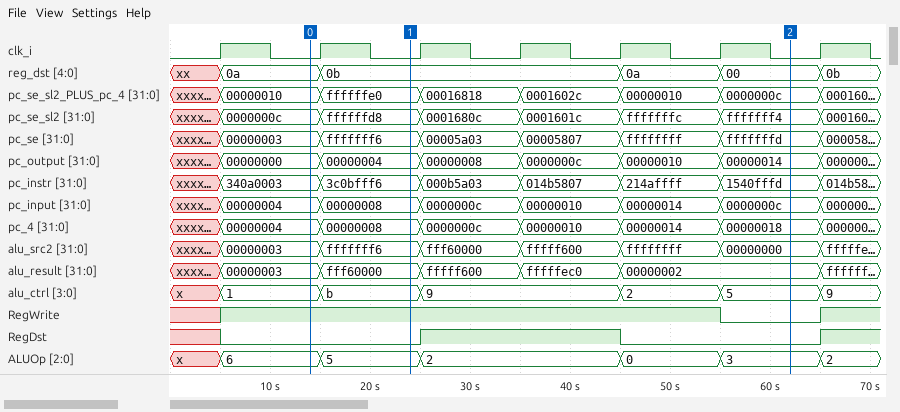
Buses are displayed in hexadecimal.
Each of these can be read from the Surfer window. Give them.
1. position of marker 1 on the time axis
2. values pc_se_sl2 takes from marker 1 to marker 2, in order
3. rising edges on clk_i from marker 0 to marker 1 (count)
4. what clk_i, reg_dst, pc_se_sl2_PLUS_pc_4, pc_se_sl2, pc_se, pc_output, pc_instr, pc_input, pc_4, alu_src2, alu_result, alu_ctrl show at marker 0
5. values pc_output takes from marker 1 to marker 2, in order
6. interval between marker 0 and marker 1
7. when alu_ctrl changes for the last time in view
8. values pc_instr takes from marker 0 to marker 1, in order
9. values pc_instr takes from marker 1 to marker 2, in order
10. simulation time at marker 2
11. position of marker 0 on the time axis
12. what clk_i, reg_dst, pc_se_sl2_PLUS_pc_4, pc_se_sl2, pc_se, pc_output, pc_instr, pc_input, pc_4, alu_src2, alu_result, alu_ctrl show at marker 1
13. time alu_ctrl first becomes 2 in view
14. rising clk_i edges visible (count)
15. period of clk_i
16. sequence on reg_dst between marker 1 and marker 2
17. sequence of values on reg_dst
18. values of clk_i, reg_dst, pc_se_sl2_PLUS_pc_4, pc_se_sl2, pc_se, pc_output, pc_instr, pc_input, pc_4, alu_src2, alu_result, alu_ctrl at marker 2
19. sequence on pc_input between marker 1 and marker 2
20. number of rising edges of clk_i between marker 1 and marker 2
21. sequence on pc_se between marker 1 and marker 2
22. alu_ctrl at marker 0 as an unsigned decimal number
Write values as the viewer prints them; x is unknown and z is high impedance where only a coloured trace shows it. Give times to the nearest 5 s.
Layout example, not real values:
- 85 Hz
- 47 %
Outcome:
- 25 s
- ffffffd8, 0001680c, 0001601c, fffffffc, fffffff4
- 1
- clk_i=0, reg_dst=0a, pc_se_sl2_PLUS_pc_4=00000010, pc_se_sl2=0000000c, pc_se=00000003, pc_output=00000000, pc_instr=340a0003, pc_input=00000004, pc_4=00000004, alu_src2=00000003, alu_result=00000003, alu_ctrl=1
- 00000004, 00000008, 0000000c, 00000010, 00000014
- 10 s
- 65 s
- 340a0003, 3c0bfff6
- 3c0bfff6, 000b5a03, 014b5807, 214affff, 1540fffd
- 60 s
- 15 s
- clk_i=0, reg_dst=0b, pc_se_sl2_PLUS_pc_4=ffffffe0, pc_se_sl2=ffffffd8, pc_se=fffffff6, pc_output=00000004, pc_instr=3c0bfff6, pc_input=00000008, pc_4=00000008, alu_src2=fffffff6, alu_result=fff60000, alu_ctrl=b
- 45 s
- 7
- 10 s
- 0b, 0a, 00
- xx, 0a, 0b, 0a, 00, 0b
- clk_i=0, reg_dst=00, pc_se_sl2_PLUS_pc_4=0000000c, pc_se_sl2=fffffff4, pc_se=fffffffd, pc_output=00000014, pc_instr=1540fffd, pc_input=0000000c, pc_4=00000018, alu_src2=00000000, alu_result=00000002, alu_ctrl=5
- 00000008, 0000000c, 00000010, 00000014, 0000000c
- 4
- fffffff6, 00005a03, 00005807, ffffffff, fffffffd
- 1
